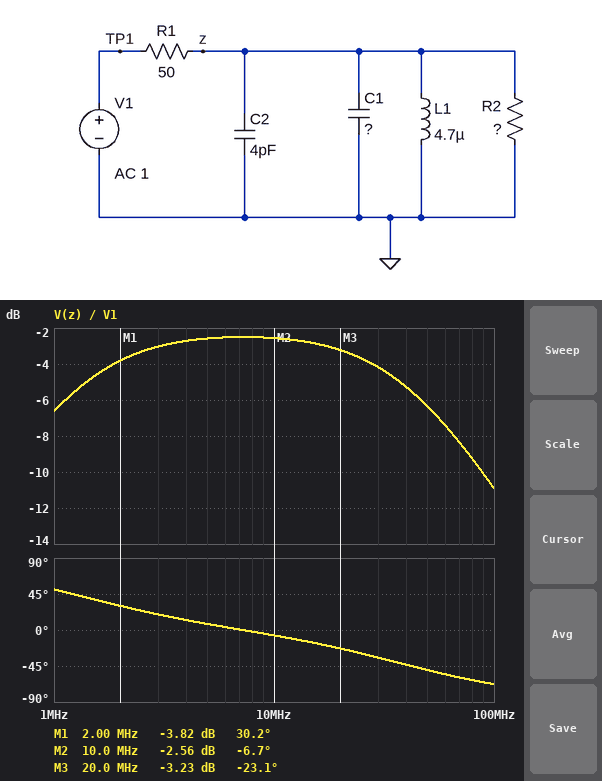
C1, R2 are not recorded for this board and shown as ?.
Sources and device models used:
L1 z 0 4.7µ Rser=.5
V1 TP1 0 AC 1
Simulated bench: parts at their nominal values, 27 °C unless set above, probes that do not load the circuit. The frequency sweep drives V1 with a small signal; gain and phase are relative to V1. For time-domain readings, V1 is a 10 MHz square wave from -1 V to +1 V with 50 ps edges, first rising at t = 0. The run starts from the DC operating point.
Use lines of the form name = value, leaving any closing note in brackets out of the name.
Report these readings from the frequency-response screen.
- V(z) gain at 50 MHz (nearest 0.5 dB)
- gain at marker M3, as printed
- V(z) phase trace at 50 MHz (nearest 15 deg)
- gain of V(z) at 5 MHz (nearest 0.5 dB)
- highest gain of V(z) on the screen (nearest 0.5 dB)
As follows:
V(z) gain at 50 MHz = -6.5 dB
gain at marker M3, as printed = -3.23 dB
V(z) phase trace at 50 MHz = -45 deg
gain of V(z) at 5 MHz = -2.5 dB
highest gain of V(z) on the screen = -2.5 dB
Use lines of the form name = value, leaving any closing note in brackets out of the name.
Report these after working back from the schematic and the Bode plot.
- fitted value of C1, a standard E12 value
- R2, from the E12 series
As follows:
fitted value of C1, a standard E12 value = 100 pF
R2, from the E12 series = 150 Ω
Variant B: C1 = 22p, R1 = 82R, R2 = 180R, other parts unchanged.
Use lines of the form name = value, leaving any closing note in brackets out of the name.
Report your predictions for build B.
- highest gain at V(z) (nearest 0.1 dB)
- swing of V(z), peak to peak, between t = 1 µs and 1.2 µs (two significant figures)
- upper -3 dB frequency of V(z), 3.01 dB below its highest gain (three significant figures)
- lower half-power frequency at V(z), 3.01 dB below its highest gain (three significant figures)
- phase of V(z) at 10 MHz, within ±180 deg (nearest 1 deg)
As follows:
highest gain at V(z) = -3.3 dB
swing of V(z), peak to peak, between t = 1 µs and 1.2 µs = 1.7 V
upper -3 dB frequency of V(z), 3.01 dB below its highest gain = 111 MHz
lower half-power frequency at V(z), 3.01 dB below its highest gain = 1.89 MHz
phase of V(z) at 10 MHz, within ±180 deg = 6 deg
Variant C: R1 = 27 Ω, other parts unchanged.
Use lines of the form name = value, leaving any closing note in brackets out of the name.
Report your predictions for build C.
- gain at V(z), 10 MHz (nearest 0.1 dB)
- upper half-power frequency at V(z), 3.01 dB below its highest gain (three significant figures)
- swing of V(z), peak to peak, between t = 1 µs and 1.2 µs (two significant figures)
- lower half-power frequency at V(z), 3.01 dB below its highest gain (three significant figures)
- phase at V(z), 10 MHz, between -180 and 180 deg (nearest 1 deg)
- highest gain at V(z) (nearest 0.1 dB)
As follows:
gain at V(z), 10 MHz = -1.5 dB
upper half-power frequency at V(z), 3.01 dB below its highest gain = 67.7 MHz
swing of V(z), peak to peak, between t = 1 µs and 1.2 µs = 1.8 V
lower half-power frequency at V(z), 3.01 dB below its highest gain = 782 kHz
phase at V(z), 10 MHz, between -180 and 180 deg = -4 deg
highest gain at V(z) = -1.4 dB
